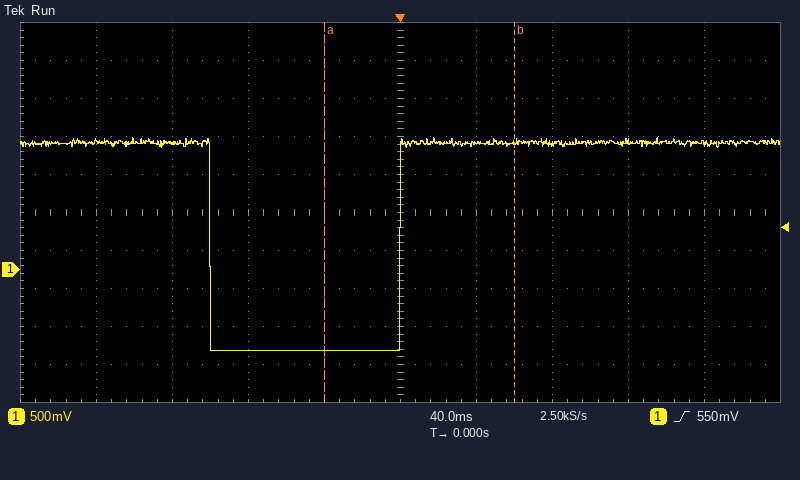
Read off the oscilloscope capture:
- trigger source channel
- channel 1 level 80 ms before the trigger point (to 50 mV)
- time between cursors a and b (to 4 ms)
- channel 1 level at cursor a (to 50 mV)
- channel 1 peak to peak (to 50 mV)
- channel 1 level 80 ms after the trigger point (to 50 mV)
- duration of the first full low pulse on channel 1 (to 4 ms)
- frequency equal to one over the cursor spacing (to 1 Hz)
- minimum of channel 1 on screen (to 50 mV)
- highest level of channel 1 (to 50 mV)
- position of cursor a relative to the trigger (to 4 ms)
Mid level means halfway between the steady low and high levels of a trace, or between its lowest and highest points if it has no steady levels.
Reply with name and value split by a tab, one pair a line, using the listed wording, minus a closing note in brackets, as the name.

trigger source channel	channel 1
channel 1 level 80 ms before the trigger point	-1.05 V
time between cursors a and b	100 ms
channel 1 level at cursor a	-1.05 V
channel 1 peak to peak	2.80 V
channel 1 level 80 ms after the trigger point	1.65 V
duration of the first full low pulse on channel 1	100 ms
frequency equal to one over the cursor spacing	10 Hz
minimum of channel 1 on screen	-1.05 V
highest level of channel 1	1.75 V
position of cursor a relative to the trigger	-40 ms
